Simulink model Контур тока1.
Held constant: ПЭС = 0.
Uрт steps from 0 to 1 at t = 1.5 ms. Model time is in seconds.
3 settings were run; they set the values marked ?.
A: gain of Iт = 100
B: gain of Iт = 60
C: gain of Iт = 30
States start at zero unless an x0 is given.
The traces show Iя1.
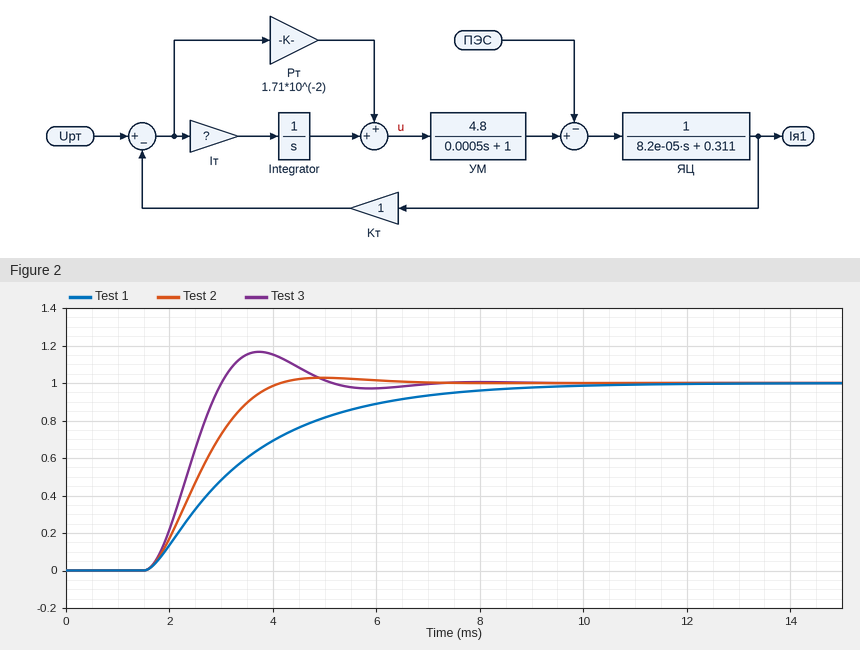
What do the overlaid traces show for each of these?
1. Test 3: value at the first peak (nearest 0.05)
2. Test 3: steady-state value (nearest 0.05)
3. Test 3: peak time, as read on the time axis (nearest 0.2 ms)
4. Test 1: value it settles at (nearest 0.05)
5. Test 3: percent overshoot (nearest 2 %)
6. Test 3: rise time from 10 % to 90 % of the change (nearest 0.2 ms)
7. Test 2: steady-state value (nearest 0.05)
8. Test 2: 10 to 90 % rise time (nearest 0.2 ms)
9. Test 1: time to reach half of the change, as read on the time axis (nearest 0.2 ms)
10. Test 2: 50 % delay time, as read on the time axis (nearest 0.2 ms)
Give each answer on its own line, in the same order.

1.15
1.00
3.8 ms
1.00
16 %
1.0 ms
1.00
1.6 ms
3.0 ms
2.6 ms
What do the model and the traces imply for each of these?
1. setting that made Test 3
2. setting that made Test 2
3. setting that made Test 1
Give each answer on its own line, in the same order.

A
B
C
